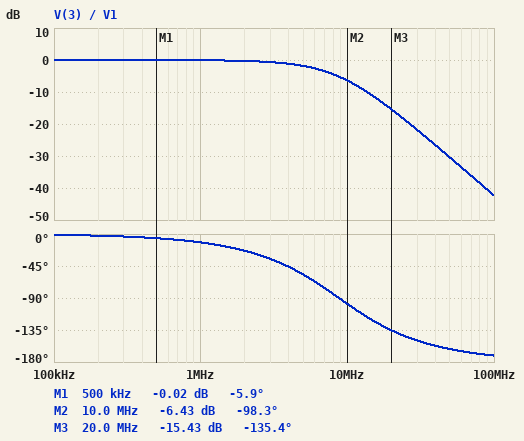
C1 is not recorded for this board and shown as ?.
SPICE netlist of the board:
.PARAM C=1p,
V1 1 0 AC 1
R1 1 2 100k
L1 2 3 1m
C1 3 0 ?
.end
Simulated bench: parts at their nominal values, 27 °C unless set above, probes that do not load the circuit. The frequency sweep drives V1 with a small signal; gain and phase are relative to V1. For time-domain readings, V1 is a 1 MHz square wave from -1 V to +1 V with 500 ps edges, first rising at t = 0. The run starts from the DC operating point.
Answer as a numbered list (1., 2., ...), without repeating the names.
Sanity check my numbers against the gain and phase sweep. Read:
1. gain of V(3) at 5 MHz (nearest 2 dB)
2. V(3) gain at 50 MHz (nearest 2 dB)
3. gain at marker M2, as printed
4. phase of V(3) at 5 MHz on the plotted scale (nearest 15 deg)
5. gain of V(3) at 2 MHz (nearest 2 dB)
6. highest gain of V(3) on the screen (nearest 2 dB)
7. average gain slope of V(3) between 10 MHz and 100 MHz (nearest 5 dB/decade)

1. -2 dB
2. -30 dB
3. -6.43 dB
4. -60 deg
5. 0 dB
6. 0 dB
7. -35 dB/decade
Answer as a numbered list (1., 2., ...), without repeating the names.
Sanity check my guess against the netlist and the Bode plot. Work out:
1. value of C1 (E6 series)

1. 330 fF
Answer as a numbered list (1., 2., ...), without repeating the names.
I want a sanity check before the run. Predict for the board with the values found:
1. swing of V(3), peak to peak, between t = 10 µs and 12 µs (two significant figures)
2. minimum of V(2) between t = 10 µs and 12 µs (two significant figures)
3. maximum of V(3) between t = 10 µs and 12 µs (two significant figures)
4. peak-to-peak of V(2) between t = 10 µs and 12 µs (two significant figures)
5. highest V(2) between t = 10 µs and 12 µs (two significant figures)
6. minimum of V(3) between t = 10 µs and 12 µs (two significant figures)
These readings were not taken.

1. 2.0 V
2. -1.0 V
3. 1.0 V
4. 2.0 V
5. 1.0 V
6. -1.0 V
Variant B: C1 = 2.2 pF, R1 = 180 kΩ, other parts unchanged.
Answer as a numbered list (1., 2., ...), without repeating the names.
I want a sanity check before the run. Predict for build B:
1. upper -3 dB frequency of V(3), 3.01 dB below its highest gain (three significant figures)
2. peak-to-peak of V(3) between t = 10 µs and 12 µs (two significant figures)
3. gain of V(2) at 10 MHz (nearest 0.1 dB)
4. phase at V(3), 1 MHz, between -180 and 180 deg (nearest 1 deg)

1. 408 kHz
2. 1.1 V
3. -10.6 dB
4. -70 deg
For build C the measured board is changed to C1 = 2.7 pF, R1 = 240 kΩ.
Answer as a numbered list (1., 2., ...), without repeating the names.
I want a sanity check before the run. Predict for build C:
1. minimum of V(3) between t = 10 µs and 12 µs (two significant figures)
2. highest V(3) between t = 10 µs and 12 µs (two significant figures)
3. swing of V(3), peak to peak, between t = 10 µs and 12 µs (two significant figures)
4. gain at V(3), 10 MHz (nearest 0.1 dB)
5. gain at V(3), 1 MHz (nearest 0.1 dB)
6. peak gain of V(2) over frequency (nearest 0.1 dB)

1. -370 mV
2. 370 mV
3. 730 mV
4. -32.4 dB
5. -12.4 dB
6. 0 dB
